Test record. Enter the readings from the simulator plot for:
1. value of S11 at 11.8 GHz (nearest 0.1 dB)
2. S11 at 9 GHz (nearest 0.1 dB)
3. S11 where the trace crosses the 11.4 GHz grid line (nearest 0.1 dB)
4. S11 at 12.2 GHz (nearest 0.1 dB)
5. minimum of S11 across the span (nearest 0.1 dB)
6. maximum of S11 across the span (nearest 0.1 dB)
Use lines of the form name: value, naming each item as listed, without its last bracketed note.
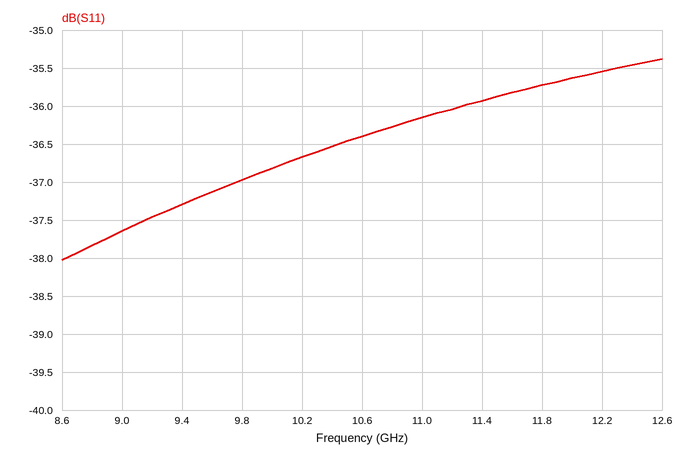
value of S11 at 11.8 GHz: -35.7 dB
S11 at 9 GHz: -37.6 dB
S11 where the trace crosses the 11.4 GHz grid line: -35.9 dB
S11 at 12.2 GHz: -35.5 dB
minimum of S11 across the span: -38.0 dB
maximum of S11 across the span: -35.4 dB
